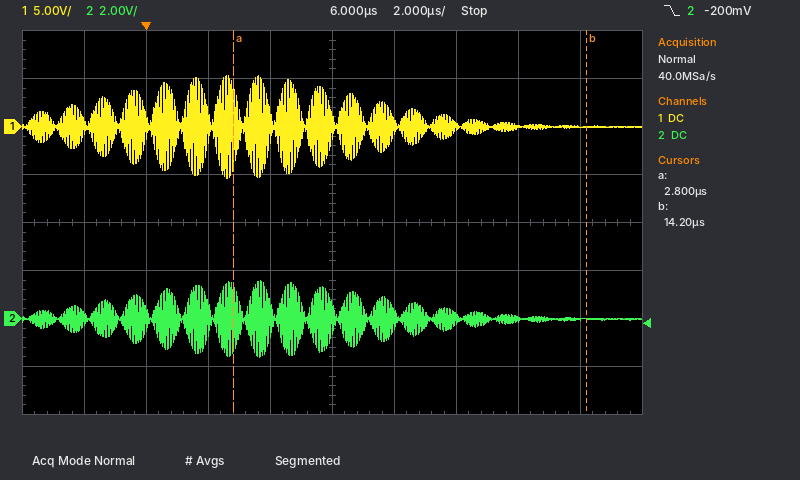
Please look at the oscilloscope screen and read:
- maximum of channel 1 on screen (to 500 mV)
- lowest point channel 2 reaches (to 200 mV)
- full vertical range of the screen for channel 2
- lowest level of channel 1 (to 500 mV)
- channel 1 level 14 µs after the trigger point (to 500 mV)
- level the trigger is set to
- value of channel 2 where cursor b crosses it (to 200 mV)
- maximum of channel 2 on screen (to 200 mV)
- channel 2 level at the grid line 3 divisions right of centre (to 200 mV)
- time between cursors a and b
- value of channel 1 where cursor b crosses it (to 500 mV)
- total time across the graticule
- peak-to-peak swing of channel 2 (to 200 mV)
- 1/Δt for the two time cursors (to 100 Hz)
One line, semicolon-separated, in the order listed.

5.5 V; -1.6 V; 16 V; -5.5 V; 0.0 V; -200 mV; 0.0 V; 1.6 V; 0.0 V; 11.4 µs; 0.0 V; 20 µs; 3.2 V; 87.7 kHz
